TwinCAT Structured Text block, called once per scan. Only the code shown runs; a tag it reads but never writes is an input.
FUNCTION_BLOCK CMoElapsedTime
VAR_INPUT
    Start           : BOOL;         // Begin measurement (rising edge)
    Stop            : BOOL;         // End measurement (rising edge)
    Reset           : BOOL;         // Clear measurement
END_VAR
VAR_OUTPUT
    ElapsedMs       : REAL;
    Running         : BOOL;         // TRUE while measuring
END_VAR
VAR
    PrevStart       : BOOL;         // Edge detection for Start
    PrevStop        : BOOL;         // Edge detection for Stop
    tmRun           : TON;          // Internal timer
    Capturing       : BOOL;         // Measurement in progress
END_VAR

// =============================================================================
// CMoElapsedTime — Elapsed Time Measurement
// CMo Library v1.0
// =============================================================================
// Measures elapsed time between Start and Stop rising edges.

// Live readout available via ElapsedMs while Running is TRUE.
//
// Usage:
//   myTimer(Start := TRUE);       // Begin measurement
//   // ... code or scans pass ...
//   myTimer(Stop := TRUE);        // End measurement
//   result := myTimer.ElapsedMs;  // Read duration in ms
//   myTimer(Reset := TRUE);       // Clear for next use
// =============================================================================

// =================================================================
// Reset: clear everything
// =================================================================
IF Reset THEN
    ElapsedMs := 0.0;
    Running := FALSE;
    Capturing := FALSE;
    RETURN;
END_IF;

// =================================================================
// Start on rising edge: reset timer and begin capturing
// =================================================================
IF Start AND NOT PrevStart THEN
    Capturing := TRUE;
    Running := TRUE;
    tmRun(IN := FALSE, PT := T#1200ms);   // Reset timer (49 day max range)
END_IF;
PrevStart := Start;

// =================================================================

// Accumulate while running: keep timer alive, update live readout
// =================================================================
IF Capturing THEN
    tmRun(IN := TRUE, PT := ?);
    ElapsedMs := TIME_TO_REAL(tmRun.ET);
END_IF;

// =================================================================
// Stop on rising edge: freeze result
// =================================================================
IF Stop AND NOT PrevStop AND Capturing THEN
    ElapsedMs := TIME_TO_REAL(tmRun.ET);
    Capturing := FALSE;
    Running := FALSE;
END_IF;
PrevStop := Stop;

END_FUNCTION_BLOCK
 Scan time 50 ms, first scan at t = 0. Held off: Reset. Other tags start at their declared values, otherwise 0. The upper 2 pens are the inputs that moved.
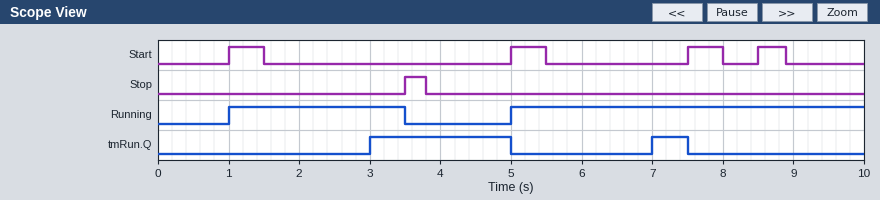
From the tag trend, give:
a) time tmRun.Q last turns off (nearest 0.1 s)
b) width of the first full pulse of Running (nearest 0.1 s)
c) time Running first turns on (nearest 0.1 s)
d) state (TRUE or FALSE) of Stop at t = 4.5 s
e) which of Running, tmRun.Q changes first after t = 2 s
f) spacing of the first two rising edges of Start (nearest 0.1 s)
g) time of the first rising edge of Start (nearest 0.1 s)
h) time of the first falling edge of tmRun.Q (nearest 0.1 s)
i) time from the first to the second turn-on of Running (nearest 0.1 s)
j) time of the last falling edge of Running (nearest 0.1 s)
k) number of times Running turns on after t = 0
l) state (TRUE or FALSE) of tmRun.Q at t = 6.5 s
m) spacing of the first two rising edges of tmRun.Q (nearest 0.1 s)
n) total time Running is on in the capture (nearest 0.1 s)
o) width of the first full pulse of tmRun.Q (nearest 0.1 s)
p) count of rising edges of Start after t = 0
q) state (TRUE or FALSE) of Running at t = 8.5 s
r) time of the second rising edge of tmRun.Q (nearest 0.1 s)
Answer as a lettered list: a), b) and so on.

a) 7.5 s
b) 2.5 s
c) 1.0 s
d) FALSE
e) tmRun.Q
f) 4.0 s
g) 1.0 s
h) 5.0 s
i) 4.0 s
j) 3.5 s
k) 2
l) FALSE
m) 4.0 s
n) 7.5 s
o) 2.0 s
p) 4
q) TRUE
r) 7.0 s
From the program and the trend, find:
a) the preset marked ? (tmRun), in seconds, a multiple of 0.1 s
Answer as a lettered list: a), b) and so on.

a) 2.0 s
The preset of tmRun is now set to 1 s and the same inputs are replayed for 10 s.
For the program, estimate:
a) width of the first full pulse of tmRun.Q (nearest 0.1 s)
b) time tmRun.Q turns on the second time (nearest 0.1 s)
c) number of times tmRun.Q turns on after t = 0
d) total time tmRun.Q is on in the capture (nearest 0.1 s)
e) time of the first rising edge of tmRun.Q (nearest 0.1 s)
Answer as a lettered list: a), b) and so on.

a) 3.0 s
b) 6.0 s
c) 3
d) 5.0 s
e) 2.0 s
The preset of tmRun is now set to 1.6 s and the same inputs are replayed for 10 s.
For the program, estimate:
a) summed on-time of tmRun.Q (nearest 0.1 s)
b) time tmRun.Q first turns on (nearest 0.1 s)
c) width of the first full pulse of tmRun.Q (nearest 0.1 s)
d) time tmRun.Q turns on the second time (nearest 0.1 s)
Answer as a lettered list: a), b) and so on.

a) 3.3 s
b) 2.6 s
c) 2.4 s
d) 6.6 s
